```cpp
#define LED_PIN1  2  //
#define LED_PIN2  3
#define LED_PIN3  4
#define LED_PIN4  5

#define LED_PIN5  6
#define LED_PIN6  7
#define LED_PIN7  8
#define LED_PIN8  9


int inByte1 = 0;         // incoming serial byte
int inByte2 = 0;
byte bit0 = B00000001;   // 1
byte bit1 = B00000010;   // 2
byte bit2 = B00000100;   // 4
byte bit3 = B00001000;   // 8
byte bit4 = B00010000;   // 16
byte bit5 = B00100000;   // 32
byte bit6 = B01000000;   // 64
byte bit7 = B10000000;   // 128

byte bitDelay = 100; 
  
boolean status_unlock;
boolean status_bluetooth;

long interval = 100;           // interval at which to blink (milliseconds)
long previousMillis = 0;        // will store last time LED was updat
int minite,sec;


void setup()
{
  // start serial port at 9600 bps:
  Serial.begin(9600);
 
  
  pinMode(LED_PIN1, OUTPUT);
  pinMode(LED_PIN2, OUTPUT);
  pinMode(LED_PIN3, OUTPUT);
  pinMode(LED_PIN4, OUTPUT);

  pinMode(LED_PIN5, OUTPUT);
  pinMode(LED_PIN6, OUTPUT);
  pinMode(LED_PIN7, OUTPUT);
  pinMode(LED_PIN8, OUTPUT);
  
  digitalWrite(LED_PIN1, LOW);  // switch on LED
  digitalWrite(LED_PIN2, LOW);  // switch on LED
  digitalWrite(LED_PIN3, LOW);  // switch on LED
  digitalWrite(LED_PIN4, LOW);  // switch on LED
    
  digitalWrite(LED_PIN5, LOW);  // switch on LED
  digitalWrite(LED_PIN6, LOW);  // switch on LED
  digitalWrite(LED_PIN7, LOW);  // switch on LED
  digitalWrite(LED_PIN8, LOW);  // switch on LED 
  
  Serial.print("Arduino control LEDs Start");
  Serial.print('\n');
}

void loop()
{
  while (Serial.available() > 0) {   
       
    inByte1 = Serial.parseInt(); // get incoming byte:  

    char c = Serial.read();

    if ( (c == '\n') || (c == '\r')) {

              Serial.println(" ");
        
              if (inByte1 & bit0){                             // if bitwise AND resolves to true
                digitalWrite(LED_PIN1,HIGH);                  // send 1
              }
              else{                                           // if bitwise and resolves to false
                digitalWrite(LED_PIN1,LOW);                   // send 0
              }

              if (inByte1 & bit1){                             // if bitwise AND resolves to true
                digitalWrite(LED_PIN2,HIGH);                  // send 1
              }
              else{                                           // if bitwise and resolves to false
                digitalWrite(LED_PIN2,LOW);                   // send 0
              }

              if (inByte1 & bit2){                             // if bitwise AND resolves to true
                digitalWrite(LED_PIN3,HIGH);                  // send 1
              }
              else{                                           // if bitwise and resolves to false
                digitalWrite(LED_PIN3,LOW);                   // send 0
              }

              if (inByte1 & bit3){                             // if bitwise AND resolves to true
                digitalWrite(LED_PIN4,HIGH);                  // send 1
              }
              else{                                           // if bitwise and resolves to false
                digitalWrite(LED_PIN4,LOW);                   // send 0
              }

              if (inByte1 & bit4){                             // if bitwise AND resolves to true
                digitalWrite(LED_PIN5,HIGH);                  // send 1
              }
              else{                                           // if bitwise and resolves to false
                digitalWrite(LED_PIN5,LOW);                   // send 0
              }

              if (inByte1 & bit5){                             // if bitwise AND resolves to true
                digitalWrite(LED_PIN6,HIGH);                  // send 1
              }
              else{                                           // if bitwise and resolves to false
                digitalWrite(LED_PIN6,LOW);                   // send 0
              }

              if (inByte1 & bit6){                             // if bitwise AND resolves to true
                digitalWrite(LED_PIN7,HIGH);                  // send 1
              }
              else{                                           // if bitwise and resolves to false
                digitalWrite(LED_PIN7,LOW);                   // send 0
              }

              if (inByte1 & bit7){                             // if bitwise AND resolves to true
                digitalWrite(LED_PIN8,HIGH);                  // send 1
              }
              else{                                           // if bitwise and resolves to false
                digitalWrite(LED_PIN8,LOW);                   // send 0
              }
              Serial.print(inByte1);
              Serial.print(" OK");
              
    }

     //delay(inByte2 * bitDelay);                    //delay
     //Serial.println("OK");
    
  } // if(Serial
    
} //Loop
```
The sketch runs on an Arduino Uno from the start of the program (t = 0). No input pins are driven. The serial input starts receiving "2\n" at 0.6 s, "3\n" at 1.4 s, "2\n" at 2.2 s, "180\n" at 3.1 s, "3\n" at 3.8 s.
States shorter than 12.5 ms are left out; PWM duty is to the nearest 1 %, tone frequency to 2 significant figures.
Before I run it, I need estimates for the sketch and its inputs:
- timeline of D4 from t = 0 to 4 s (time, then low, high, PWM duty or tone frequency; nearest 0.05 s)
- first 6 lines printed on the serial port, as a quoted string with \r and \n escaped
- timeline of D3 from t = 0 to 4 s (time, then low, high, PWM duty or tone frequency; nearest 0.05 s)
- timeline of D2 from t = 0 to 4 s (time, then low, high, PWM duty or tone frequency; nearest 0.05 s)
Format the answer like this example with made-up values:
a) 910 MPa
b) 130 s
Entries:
a) 0 s low; 3.1 s high; 3.8 s low
b) "Arduino control LEDs Start\n \r\n2 OK \r\n3 OK \r\n2 OK \r\n180 OK \r\n"
c) 0 s low; 0.6 s high; 3.1 s low; 3.8 s high
d) 0 s low; 1.4 s high; 2.2 s low; 3.8 s high
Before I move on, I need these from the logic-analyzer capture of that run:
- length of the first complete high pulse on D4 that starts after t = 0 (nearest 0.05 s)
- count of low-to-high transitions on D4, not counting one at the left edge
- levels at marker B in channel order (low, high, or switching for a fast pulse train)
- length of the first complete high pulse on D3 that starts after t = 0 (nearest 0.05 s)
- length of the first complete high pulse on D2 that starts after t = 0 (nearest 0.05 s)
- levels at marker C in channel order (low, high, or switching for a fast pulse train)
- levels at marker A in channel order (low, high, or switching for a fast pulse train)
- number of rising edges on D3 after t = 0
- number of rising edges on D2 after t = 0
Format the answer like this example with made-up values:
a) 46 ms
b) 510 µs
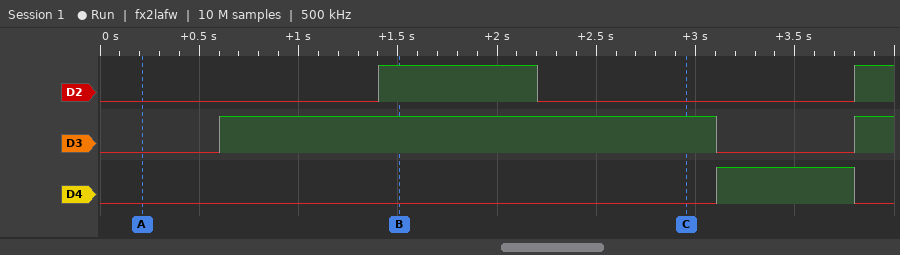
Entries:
a) 0.70 s
b) 1
c) D2 high, D3 high, D4 low
d) 2.50 s
e) 0.80 s
f) D2 low, D3 high, D4 low
g) D2 low, D3 low, D4 low
h) 2
i) 2
